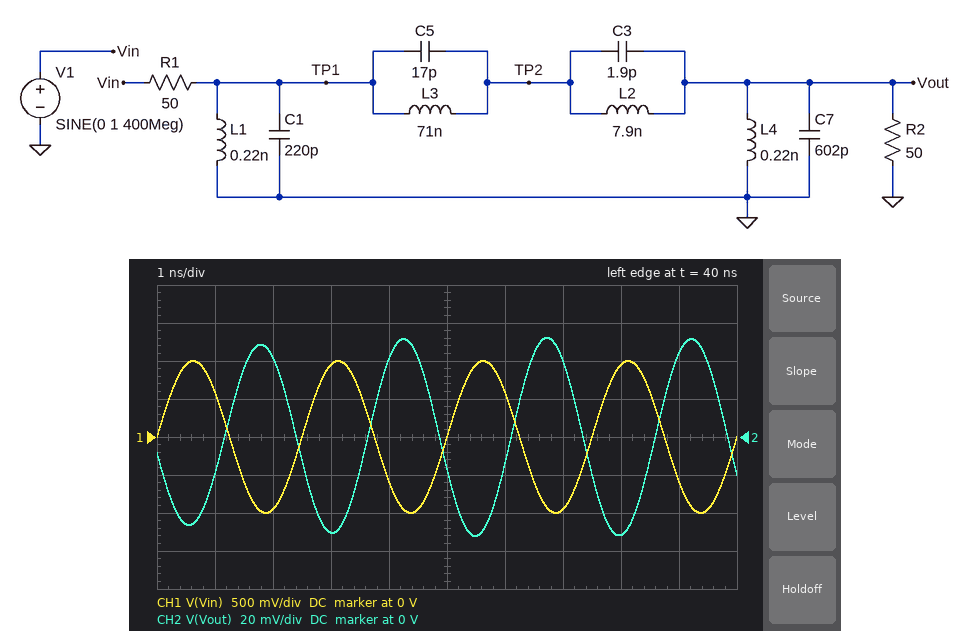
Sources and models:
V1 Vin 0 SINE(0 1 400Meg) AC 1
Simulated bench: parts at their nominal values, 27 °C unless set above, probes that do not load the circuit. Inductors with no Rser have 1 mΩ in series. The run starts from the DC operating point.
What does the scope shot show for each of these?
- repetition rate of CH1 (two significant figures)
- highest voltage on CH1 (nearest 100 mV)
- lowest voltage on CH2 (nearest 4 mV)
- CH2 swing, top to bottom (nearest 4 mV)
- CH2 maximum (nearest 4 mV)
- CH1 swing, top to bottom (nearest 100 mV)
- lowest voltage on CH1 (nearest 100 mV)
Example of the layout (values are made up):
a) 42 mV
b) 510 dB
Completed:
a) 400 MHz
b) 1.0 V
c) -52 mV
d) 104 mV
e) 52 mV
f) 2.0 V
g) -1.0 V
